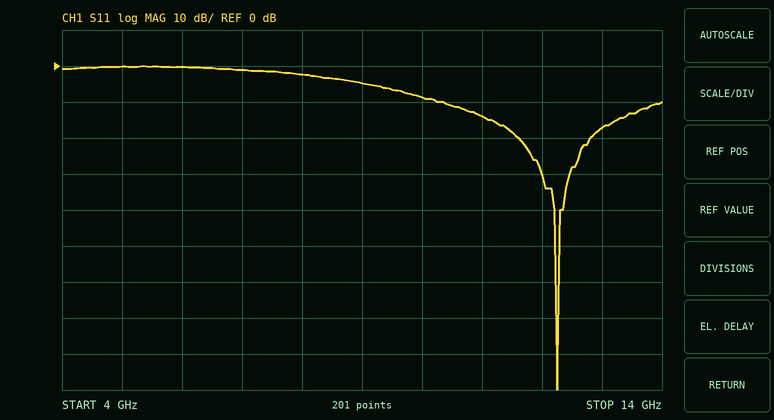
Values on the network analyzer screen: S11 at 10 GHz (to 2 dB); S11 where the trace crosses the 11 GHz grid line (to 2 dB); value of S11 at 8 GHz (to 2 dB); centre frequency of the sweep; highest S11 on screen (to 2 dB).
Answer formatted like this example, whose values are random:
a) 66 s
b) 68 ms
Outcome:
a) -8 dB
b) -14 dB
c) -2 dB
d) 9 GHz
e) 0 dB
